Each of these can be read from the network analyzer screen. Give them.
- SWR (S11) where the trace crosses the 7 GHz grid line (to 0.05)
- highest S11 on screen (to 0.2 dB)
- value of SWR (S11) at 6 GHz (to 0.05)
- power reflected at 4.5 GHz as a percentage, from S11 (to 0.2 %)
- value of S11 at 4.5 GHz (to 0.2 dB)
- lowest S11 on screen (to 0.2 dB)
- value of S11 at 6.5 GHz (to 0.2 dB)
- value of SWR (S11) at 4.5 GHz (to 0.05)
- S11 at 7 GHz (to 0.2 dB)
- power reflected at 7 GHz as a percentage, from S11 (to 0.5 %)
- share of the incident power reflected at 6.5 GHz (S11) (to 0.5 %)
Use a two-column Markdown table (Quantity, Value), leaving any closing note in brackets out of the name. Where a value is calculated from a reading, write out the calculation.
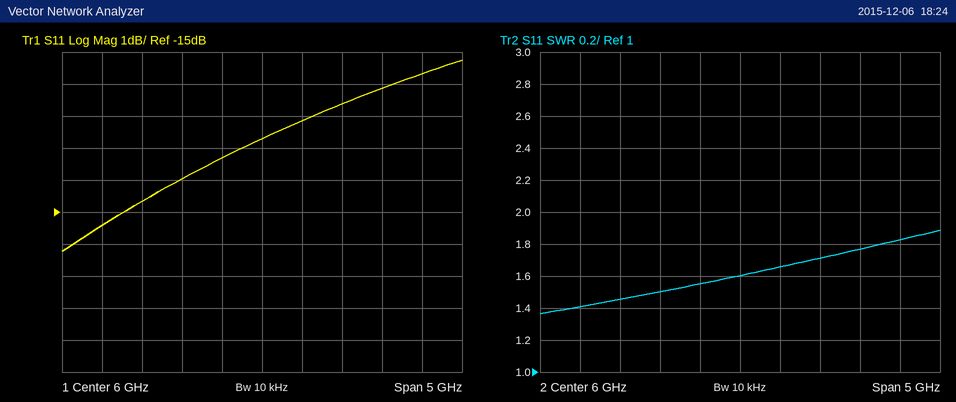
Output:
| Quantity | Value |
|---|---|
| SWR (S11) where the trace crosses the 7 GHz grid line | 1.70 |
| highest S11 on screen | -10.2 dB |
| value of SWR (S11) at 6 GHz | 1.60 |
| power reflected at 4.5 GHz as a percentage, from S11 | 10^(-14.6/10) ≈ 3.47 %, so 3.4 % to the nearest 0.2 % |
| value of S11 at 4.5 GHz | -14.6 dB |
| lowest S11 on screen | -16.2 dB |
| value of S11 at 6.5 GHz | -12.2 dB |
| value of SWR (S11) at 4.5 GHz | 1.45 |
| S11 at 7 GHz | -11.6 dB |
| power reflected at 7 GHz as a percentage, from S11 | 10^(-11.6/10) ≈ 6.92 %, so 7.0 % to the nearest 0.5 % |
| share of the incident power reflected at 6.5 GHz (S11) | 10^(-12.2/10) ≈ 6.0 % |
